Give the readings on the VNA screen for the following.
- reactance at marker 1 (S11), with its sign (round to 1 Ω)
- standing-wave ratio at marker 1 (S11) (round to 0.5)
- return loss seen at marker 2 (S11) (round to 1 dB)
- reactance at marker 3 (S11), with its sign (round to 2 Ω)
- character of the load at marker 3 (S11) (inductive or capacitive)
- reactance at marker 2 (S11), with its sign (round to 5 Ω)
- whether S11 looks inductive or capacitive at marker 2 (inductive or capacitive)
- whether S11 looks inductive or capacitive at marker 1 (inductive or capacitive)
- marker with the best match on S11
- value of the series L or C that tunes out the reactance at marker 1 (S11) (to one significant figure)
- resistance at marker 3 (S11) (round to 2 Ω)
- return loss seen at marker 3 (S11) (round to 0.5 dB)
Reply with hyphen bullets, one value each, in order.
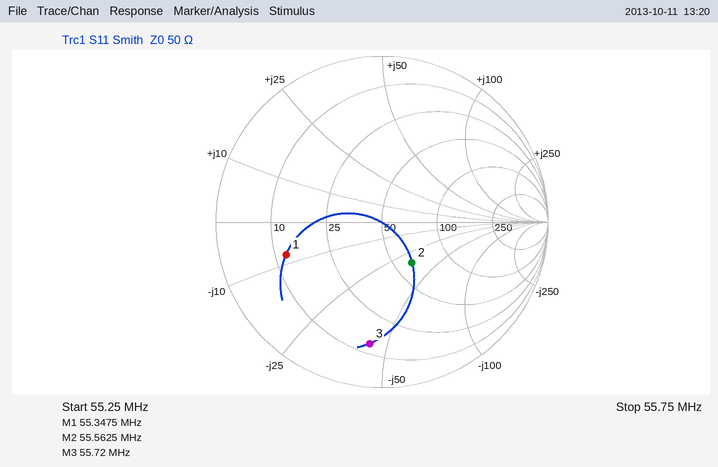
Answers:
- -8 Ω
- 4.0
- 10 dB
- -44 Ω
- capacitive
- -35 Ω
- capacitive
- capacitive
- marker 2
- 20 nH
- 14 Ω
- 2.5 dB
